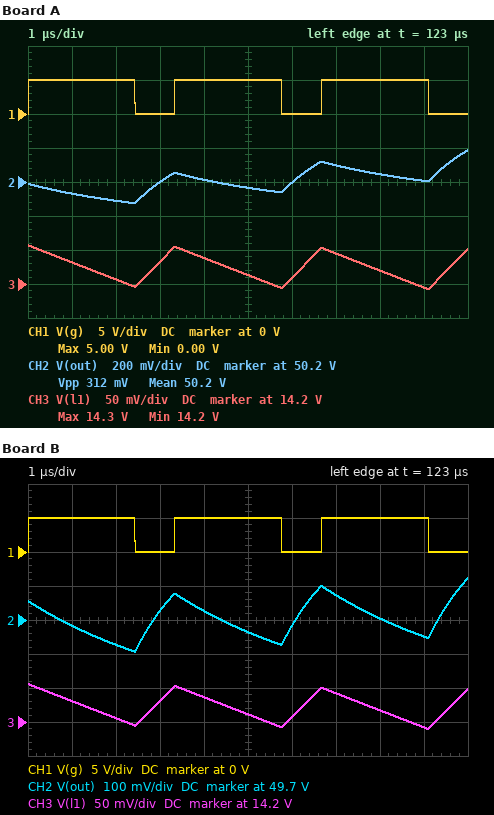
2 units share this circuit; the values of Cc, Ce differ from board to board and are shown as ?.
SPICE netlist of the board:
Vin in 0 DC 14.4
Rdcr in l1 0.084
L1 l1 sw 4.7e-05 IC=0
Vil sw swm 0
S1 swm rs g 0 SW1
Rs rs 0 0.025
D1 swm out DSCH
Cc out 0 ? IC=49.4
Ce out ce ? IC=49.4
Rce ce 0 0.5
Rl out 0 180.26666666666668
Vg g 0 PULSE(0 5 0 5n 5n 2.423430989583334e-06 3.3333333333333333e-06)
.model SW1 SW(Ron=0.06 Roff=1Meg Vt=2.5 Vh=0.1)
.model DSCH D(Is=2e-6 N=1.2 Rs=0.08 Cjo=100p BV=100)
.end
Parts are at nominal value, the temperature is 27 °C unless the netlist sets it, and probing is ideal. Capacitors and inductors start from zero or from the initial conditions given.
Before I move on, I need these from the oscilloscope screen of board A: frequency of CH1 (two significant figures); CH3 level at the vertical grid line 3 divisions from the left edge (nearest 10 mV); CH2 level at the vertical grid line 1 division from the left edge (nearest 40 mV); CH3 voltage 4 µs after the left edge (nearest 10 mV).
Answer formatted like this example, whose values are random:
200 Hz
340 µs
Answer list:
300 kHz
14.23 V
50.12 V
14.24 V
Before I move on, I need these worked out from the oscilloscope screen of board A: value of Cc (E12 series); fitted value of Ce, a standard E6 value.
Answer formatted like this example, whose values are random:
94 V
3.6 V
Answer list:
8.2 µF
6.8 µF
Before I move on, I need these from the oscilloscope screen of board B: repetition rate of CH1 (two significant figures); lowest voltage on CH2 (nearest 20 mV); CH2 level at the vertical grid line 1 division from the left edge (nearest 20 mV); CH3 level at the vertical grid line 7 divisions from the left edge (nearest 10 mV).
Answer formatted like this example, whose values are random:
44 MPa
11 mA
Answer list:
300 kHz
49.60 V
49.68 V
14.24 V
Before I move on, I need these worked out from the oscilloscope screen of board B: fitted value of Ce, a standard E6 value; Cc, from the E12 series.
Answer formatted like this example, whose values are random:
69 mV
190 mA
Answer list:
47 µF
8.2 µF
